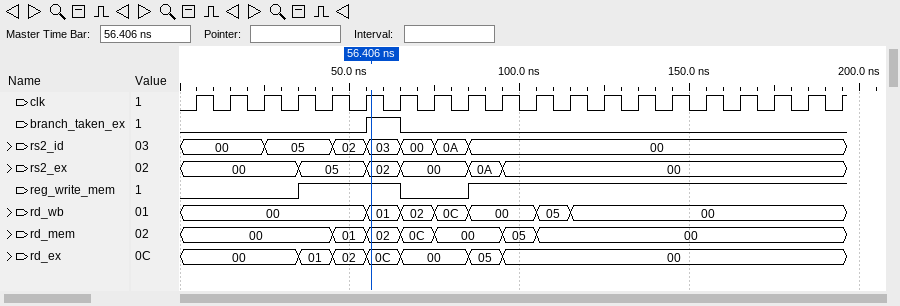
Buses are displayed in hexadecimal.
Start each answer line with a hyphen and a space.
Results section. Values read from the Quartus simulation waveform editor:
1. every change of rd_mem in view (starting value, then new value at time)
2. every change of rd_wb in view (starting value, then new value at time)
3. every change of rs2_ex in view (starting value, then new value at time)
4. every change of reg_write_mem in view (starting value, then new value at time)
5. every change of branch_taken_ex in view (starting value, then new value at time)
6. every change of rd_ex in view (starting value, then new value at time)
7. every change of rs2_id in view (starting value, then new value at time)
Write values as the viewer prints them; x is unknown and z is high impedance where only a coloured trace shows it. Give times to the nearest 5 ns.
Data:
- 00, 01 at 45 ns, 02 at 55 ns, 0C at 65 ns, 00 at 75 ns, 05 at 95 ns, 00 at 105 ns
- 00, 01 at 55 ns, 02 at 65 ns, 0C at 75 ns, 00 at 85 ns, 05 at 105 ns, 00 at 115 ns
- 00, 05 at 35 ns, 02 at 55 ns, 00 at 65 ns, 0A at 85 ns, 00 at 95 ns
- 0, 1 at 35 ns, 0 at 65 ns, 1 at 85 ns
- 0, 1 at 55 ns, 0 at 65 ns
- 00, 01 at 35 ns, 02 at 45 ns, 0C at 55 ns, 00 at 65 ns, 05 at 85 ns, 00 at 95 ns
- 00, 05 at 25 ns, 02 at 45 ns, 03 at 55 ns, 00 at 65 ns, 0A at 75 ns, 00 at 85 ns
